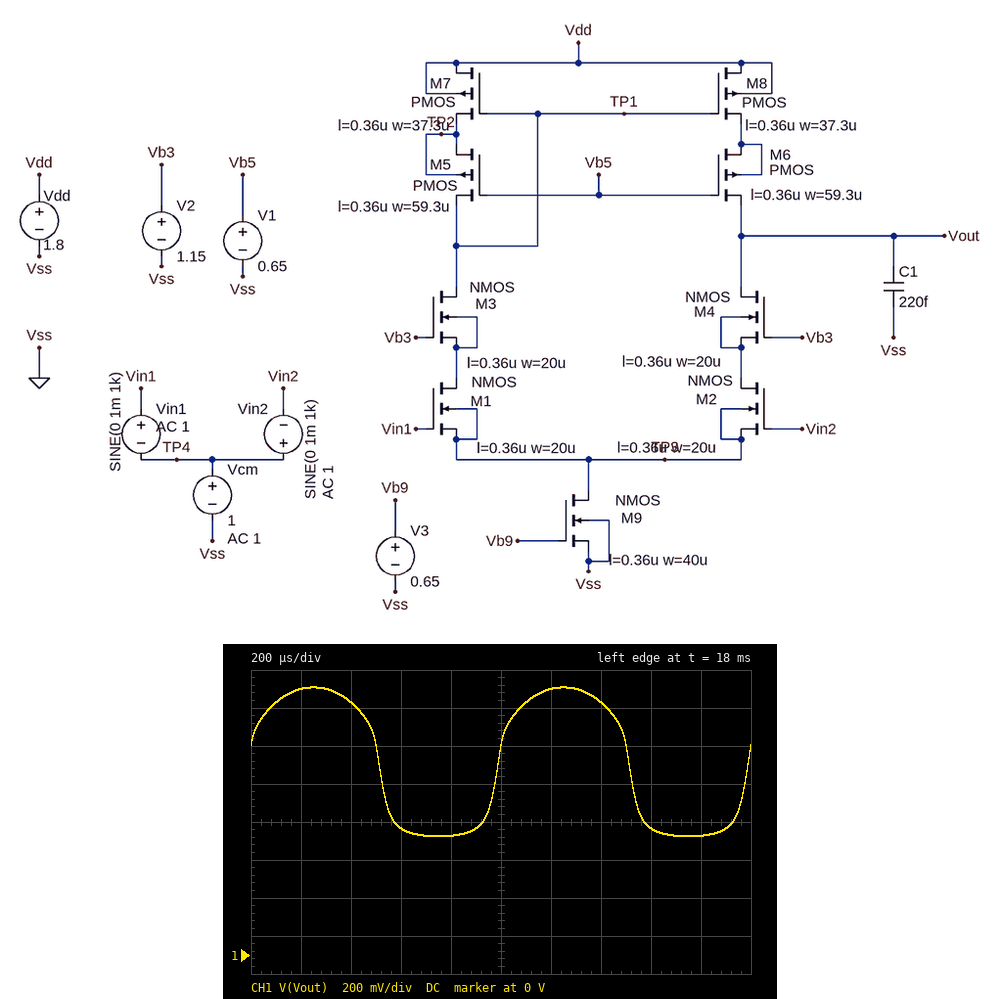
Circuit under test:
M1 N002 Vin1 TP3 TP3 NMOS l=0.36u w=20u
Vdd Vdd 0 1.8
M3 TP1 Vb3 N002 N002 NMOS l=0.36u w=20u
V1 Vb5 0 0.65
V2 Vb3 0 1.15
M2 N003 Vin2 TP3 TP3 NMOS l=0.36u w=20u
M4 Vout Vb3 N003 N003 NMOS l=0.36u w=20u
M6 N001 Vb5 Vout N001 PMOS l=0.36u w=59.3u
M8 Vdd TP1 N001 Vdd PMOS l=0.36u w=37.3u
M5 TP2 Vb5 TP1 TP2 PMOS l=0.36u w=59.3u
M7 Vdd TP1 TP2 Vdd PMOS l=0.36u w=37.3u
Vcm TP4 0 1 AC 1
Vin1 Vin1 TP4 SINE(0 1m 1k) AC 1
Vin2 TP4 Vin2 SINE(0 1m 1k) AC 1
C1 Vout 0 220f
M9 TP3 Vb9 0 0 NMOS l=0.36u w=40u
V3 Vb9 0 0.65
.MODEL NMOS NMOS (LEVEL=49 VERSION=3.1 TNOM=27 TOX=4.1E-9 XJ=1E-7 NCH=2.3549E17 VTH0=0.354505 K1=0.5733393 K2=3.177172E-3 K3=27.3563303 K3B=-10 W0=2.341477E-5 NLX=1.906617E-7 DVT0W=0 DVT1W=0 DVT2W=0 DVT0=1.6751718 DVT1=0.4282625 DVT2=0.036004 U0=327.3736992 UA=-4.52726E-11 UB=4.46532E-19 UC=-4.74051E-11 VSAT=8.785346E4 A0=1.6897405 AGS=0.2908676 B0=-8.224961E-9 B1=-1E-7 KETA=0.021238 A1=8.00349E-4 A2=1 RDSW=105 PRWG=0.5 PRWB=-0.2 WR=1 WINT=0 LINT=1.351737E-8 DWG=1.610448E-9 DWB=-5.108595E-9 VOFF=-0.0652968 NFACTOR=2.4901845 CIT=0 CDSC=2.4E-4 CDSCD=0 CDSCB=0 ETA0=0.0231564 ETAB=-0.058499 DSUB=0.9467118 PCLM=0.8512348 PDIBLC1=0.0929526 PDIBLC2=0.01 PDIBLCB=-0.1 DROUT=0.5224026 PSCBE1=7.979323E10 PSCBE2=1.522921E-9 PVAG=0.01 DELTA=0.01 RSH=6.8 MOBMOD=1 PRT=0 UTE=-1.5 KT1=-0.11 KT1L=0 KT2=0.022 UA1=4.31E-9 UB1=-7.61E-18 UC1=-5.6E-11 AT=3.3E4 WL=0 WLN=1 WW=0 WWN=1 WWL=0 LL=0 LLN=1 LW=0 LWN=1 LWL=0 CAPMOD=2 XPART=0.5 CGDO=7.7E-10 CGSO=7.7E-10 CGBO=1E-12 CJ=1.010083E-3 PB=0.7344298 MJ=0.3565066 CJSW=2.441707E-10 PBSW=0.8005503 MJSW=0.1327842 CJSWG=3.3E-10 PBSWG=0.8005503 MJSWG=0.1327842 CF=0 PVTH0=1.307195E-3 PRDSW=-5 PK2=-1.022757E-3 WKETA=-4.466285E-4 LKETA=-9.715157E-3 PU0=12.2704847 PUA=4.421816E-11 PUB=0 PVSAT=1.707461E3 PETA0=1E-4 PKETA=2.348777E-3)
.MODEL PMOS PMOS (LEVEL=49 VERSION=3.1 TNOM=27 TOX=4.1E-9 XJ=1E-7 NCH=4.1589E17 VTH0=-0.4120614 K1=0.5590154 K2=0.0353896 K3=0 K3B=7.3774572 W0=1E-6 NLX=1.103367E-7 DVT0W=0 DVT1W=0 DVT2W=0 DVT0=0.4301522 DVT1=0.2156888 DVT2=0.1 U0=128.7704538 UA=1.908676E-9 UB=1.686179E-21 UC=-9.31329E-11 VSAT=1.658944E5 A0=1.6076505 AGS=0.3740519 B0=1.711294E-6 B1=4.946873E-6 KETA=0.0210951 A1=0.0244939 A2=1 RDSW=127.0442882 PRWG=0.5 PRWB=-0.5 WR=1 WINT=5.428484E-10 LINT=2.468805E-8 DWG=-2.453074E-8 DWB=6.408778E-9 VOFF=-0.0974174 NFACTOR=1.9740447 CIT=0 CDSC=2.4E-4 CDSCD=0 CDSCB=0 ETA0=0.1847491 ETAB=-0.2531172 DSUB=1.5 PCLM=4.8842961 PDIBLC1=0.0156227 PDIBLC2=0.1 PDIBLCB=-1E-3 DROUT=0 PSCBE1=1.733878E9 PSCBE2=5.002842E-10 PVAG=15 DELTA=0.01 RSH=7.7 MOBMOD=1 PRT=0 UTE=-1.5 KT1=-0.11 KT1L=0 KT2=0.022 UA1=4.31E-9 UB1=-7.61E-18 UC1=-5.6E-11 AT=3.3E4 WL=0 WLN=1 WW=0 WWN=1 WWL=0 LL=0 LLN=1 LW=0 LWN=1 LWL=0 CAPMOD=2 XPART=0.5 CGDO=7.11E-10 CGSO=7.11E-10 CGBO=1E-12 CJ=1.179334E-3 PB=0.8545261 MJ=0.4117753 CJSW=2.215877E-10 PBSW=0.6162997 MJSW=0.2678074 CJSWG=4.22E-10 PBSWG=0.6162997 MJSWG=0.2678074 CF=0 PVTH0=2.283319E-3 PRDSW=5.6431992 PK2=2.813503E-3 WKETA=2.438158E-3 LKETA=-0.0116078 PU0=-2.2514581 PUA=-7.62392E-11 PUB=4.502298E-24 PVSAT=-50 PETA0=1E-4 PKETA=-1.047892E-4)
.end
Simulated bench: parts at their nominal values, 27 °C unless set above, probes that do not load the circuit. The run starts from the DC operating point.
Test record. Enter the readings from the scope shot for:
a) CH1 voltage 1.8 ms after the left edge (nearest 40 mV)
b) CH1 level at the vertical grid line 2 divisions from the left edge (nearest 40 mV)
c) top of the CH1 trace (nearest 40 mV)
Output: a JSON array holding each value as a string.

["640 mV", "1.32 V", "1.40 V"]
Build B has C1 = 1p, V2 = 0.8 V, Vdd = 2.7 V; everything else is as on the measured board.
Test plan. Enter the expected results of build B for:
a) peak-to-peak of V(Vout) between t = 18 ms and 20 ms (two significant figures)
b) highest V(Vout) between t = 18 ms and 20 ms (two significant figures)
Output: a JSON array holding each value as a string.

["20 mV", "2.0 V"]
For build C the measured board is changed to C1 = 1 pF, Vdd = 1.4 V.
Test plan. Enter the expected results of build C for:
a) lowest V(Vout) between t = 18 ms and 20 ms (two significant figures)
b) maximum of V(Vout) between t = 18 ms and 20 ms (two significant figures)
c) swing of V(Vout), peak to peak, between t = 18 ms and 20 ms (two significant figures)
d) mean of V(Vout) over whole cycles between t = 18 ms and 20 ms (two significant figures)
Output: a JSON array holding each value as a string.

["590 mV", "850 mV", "260 mV", "680 mV"]
